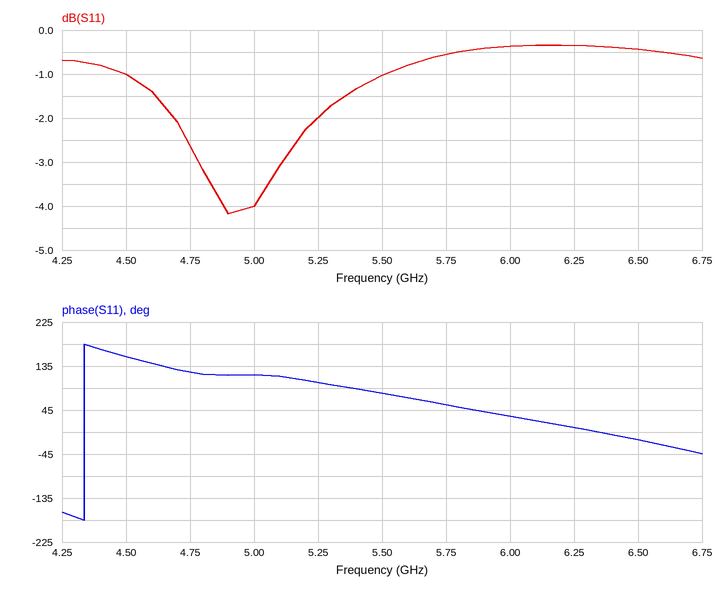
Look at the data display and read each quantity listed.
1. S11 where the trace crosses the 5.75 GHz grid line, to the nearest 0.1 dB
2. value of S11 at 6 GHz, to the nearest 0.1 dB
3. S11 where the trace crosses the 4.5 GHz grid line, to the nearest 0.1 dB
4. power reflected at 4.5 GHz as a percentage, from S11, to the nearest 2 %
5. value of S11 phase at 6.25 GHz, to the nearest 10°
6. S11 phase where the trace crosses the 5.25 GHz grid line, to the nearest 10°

-0.6 dB
-0.4 dB
-1.0 dB
80 %
10°
100°
